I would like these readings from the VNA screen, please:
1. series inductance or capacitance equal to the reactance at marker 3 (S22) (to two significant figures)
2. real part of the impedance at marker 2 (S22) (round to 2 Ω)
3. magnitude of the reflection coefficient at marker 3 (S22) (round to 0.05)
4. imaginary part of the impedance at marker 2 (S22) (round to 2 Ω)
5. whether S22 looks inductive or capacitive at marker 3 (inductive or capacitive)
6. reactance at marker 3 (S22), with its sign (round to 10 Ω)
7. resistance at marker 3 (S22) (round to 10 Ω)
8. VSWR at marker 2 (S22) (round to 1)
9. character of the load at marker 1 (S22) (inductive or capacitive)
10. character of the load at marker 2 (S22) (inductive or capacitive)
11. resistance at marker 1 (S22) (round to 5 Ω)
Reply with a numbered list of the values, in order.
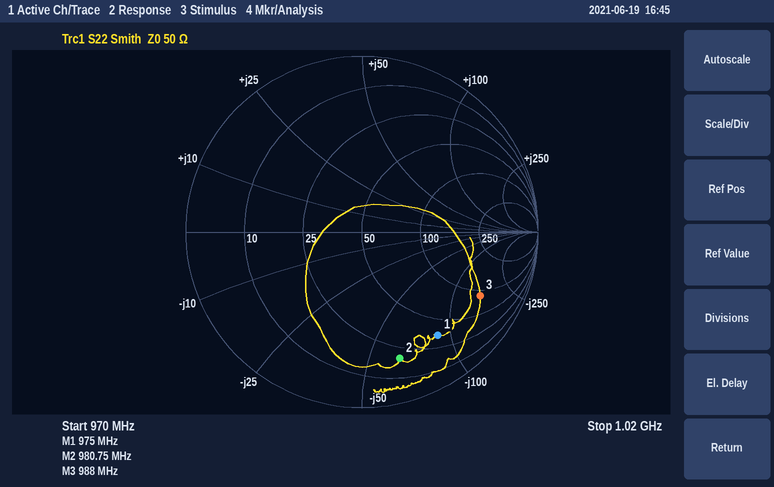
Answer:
1. 1.1 pF
2. 20 Ω
3. 0.75
4. -64 Ω
5. capacitive
6. -150 Ω
7. 90 Ω
8. 7
9. capacitive
10. capacitive
11. 35 Ω
